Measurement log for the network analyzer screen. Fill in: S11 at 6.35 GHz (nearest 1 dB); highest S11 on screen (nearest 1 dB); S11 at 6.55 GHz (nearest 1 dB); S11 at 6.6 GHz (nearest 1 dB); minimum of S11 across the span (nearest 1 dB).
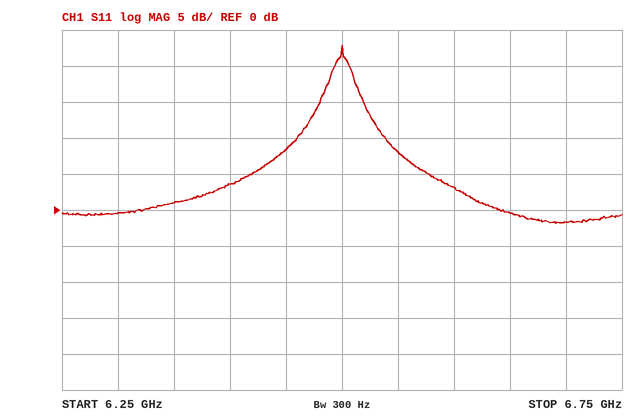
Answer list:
1 dB
23 dB
8 dB
3 dB
-2 dB
